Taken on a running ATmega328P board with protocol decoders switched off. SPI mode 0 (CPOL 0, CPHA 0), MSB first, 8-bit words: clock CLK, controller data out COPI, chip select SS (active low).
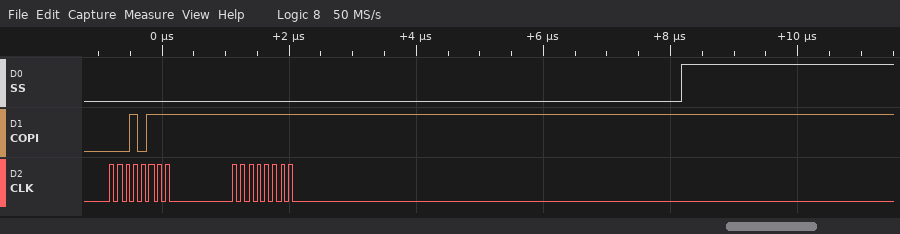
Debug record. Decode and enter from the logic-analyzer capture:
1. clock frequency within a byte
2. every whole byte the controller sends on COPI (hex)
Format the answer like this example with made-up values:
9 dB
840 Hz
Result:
8 MHz
0x17 0xFF
